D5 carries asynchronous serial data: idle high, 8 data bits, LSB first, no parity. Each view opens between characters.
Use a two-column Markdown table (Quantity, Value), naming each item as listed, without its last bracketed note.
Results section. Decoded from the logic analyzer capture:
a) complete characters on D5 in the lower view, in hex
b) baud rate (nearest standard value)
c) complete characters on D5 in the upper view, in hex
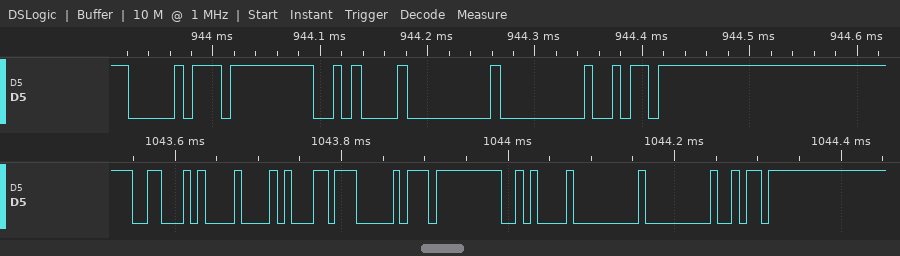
| Quantity | Value |
|---|---|
| complete characters on D5 in the lower view, in hex | 46, 08, B1, D0, FF, 0A, 00, 00, DA |
| baud rate | 115200 baud |
| complete characters on D5 in the upper view, in hex | D0, FF, 0A, 00, 00, DA |
